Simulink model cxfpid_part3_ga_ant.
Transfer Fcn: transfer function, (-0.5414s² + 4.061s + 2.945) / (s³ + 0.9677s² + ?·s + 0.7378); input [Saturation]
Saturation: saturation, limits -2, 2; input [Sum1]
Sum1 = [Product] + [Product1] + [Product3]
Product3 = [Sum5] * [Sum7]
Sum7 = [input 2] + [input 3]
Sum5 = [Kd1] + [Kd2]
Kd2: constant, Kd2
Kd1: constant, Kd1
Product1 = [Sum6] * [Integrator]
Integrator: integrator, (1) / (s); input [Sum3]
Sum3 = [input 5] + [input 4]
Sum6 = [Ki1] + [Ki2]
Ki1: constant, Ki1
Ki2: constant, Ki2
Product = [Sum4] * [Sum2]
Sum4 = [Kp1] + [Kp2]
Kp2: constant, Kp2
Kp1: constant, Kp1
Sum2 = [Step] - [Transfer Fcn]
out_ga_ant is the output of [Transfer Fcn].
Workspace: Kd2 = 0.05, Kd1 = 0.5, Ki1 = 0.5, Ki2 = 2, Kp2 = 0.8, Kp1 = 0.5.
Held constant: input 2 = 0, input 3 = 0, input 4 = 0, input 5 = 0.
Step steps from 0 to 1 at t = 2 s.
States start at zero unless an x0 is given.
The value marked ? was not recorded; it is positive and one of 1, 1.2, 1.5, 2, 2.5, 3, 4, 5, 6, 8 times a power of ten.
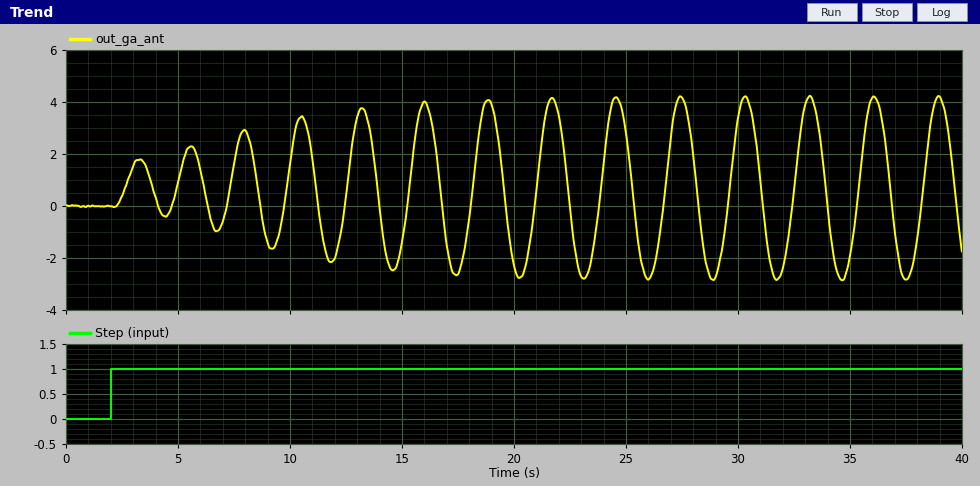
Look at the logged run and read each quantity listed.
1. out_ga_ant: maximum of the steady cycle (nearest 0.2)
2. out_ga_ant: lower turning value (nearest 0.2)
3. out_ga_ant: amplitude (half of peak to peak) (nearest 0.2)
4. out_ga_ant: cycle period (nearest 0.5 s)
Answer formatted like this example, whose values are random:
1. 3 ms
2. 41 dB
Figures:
1. 4.2
2. -2.8
3. 3.6
4. 3.0 s
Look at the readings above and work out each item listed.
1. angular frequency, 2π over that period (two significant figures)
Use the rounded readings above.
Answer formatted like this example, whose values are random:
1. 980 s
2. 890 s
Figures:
1. 2.1 rad/s
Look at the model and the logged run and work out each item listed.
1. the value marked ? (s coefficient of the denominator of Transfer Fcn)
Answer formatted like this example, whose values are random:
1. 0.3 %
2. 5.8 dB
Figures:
1. 2
